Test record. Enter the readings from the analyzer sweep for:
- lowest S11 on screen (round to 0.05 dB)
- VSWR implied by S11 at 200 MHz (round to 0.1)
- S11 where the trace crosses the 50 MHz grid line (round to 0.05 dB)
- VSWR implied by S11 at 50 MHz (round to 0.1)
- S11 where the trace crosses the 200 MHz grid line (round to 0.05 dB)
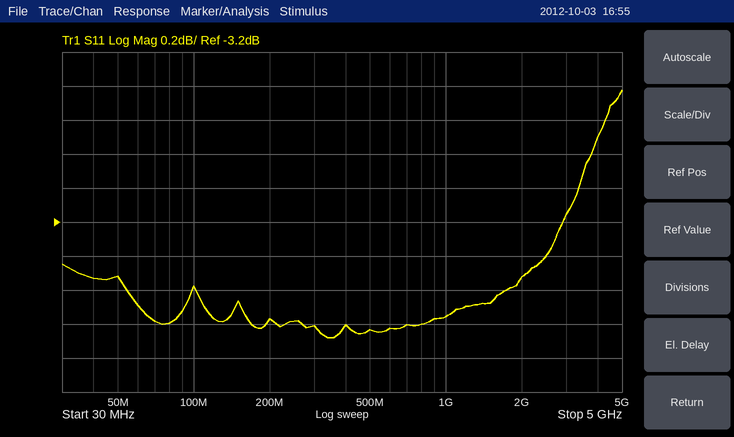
-3.90 dB
4.7
-3.50 dB
5.0
-3.75 dB
